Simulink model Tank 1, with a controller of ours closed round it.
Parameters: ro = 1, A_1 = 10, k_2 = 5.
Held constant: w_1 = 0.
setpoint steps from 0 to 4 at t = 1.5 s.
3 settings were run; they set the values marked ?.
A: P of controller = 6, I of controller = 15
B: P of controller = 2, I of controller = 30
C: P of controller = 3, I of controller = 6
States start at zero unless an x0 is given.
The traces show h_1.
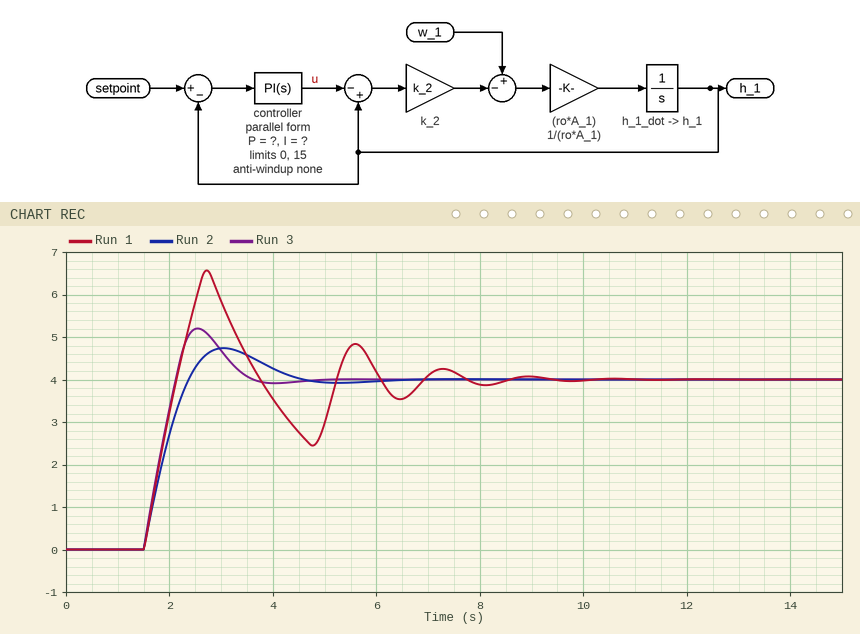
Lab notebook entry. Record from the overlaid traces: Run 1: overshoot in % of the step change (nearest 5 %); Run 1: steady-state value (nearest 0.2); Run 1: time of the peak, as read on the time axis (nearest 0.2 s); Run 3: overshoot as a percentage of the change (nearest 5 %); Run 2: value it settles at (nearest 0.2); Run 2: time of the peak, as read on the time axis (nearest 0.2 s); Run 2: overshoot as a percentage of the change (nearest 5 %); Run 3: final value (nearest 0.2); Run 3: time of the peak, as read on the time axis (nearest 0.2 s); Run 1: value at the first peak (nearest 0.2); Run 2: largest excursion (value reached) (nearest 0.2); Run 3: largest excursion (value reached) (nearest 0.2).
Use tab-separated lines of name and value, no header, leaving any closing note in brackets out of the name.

Run 1: overshoot in % of the step change	65 %
Run 1: steady-state value	4.0
Run 1: time of the peak, as read on the time axis	2.8 s
Run 3: overshoot as a percentage of the change	30 %
Run 2: value it settles at	4.0
Run 2: time of the peak, as read on the time axis	3.0 s
Run 2: overshoot as a percentage of the change	20 %
Run 3: final value	4.0
Run 3: time of the peak, as read on the time axis	2.6 s
Run 1: value at the first peak	6.6
Run 2: largest excursion (value reached)	4.8
Run 3: largest excursion (value reached)	5.2
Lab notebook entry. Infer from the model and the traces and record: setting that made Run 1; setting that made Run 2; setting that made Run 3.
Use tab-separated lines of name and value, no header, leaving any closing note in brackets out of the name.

setting that made Run 1	B
setting that made Run 2	C
setting that made Run 3	A
